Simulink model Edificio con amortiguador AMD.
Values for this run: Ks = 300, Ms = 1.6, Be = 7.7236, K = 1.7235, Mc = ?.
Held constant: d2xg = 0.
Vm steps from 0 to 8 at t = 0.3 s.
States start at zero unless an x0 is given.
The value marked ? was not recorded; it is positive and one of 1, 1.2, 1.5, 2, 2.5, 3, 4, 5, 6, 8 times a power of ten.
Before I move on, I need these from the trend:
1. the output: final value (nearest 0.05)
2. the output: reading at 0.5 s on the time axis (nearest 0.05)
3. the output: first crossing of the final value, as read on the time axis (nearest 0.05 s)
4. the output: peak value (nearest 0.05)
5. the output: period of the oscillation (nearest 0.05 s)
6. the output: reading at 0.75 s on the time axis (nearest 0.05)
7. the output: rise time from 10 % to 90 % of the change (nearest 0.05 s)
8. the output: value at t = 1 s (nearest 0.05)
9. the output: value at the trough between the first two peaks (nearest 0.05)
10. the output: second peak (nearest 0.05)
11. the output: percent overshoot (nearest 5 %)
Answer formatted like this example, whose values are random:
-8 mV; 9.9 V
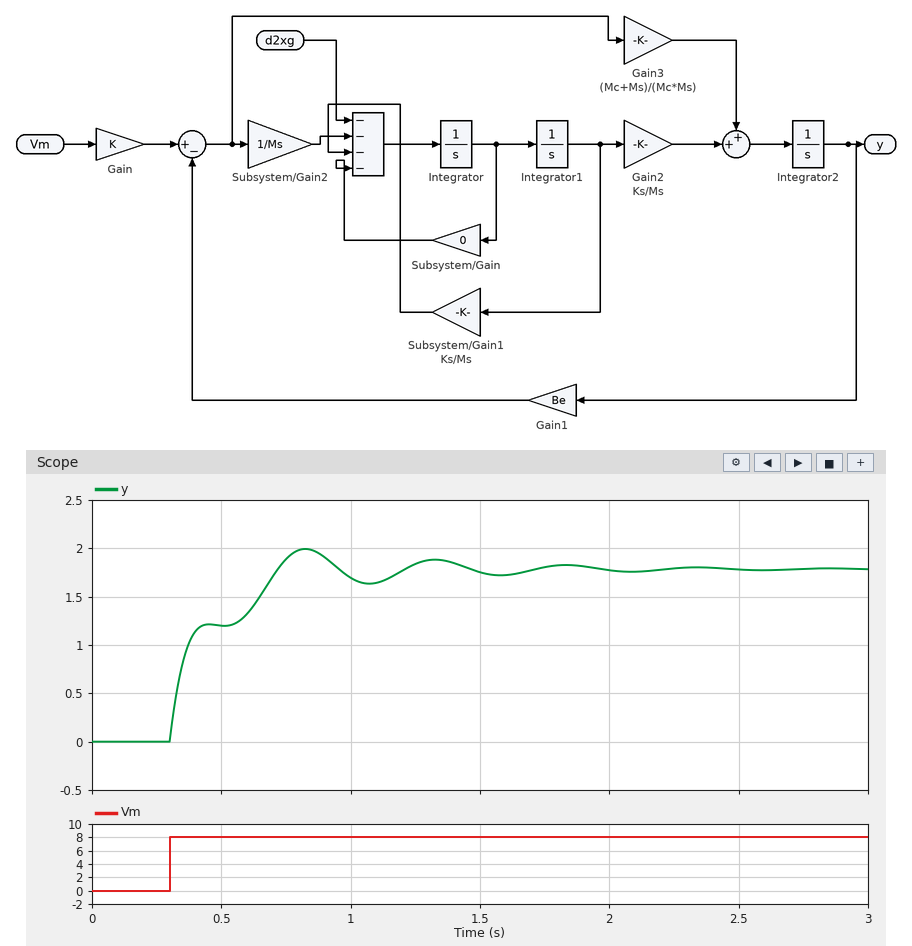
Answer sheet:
1.80; 1.20; 0.70 s; 2.00; 0.50 s; 1.90; 0.35 s; 1.70; 1.65; 1.90; 10 %
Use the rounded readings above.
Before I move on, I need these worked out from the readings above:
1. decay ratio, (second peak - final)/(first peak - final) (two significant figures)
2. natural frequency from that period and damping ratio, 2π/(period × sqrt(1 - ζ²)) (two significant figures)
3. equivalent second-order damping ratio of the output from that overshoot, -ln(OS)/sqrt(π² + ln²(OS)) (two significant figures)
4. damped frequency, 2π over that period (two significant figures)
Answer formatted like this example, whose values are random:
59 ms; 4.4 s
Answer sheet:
0.50; 16 rad/s; 0.59; 13 rad/s
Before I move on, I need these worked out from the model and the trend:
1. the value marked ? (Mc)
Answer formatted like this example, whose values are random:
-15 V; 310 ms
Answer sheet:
1
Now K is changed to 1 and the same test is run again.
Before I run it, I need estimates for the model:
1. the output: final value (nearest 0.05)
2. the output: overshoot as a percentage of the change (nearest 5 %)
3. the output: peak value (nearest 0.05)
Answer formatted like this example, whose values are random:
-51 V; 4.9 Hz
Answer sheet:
1.05; 10 %; 1.15
